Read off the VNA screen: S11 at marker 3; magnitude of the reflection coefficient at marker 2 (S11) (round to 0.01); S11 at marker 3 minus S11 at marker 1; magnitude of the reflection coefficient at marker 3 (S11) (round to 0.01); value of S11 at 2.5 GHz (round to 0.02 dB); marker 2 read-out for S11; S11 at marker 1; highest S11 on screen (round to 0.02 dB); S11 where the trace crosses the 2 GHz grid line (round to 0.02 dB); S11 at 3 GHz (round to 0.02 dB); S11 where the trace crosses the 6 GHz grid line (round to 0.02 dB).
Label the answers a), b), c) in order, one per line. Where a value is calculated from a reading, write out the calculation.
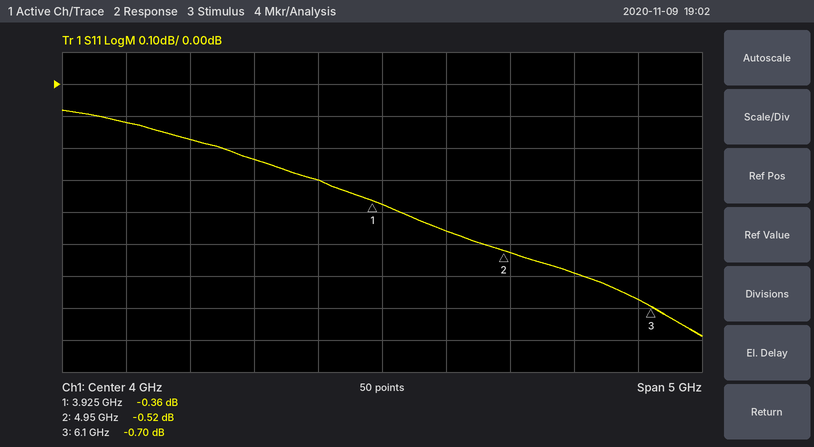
a) -0.70 dB
b) 10^(-0.52/20) ≈ 0.94
c) -0.7 − (-0.36) = -0.34 dB
d) 10^(-0.7/20) ≈ 0.92
e) -0.18 dB
f) -0.52 dB
g) -0.36 dB
h) -0.08 dB
i) -0.12 dB
j) -0.24 dB
k) -0.68 dB
